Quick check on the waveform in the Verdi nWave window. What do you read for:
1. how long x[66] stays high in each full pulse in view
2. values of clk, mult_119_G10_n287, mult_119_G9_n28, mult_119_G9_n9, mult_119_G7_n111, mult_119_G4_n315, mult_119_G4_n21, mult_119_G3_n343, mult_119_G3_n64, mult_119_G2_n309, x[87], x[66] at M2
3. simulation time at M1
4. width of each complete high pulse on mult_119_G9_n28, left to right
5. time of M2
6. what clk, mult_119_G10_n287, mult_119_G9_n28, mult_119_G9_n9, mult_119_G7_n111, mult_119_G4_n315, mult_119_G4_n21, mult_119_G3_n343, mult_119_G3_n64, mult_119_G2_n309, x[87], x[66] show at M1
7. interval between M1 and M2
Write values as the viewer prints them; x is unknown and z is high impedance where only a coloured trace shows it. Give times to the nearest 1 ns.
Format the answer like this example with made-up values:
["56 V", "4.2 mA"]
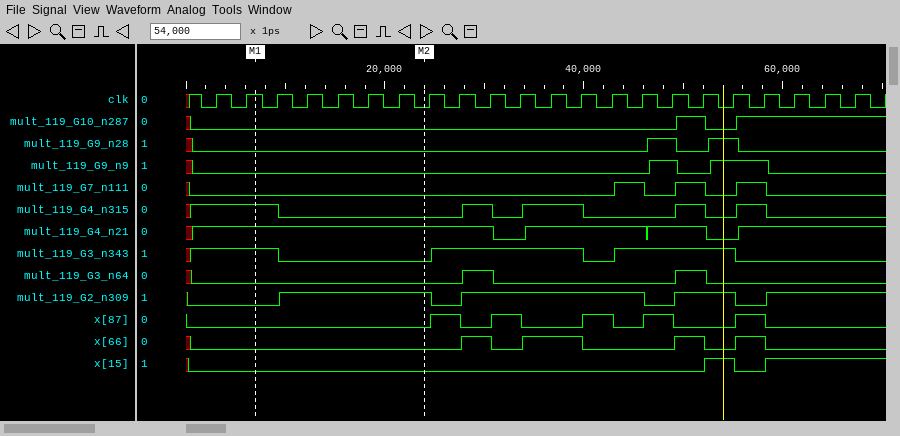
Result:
["3 ns, 6 ns, 3 ns, 3 ns", "clk=0, mult_119_G10_n287=0, mult_119_G9_n28=0, mult_119_G9_n9=0, mult_119_G7_n111=0, mult_119_G4_n315=0, mult_119_G4_n21=1, mult_119_G3_n343=0, mult_119_G3_n64=0, mult_119_G2_n309=1, x[87]=0, x[66]=0", "7 ns", "3 ns, 3 ns", "24 ns", "clk=1, mult_119_G10_n287=0, mult_119_G9_n28=0, mult_119_G9_n9=0, mult_119_G7_n111=0, mult_119_G4_n315=1, mult_119_G4_n21=1, mult_119_G3_n343=1, mult_119_G3_n64=0, mult_119_G2_n309=0, x[87]=0, x[66]=0", "17 ns"]
